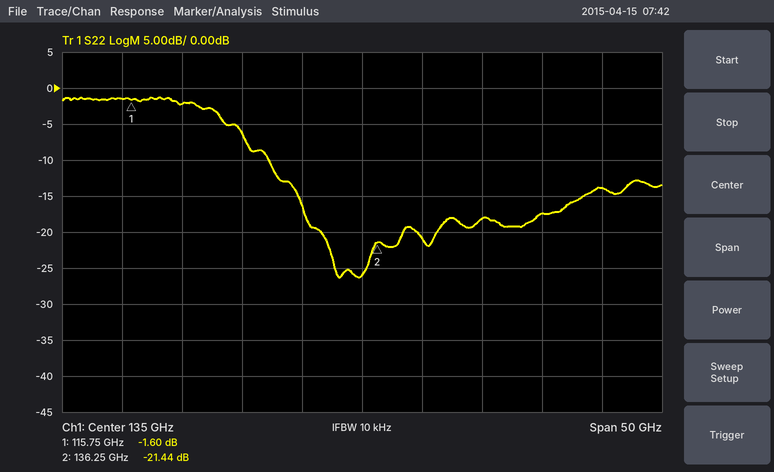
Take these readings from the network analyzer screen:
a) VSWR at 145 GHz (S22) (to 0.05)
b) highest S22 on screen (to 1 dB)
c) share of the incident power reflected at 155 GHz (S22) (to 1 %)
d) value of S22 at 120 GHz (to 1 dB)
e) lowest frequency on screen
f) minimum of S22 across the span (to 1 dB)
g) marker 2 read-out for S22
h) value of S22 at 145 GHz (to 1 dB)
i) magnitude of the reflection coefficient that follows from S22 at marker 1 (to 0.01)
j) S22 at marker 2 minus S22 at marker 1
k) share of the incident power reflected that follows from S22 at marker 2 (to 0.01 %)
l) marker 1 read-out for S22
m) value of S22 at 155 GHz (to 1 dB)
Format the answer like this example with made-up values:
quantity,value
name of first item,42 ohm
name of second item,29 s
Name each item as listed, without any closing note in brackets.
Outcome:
quantity,value
VSWR at 145 GHz (S22),1.30
highest S22 on screen,-1 dB
share of the incident power reflected at 155 GHz (S22),4 %
value of S22 at 120 GHz,-2 dB
lowest frequency on screen,110 GHz
minimum of S22 across the span,-26 dB
marker 2 read-out for S22,-21.44 dB
value of S22 at 145 GHz,-18 dB
magnitude of the reflection coefficient that follows from S22 at marker 1,0.83
S22 at marker 2 minus S22 at marker 1,-19.84 dB
share of the incident power reflected that follows from S22 at marker 2,0.72 %
marker 1 read-out for S22,-1.60 dB
value of S22 at 155 GHz,-14 dB
